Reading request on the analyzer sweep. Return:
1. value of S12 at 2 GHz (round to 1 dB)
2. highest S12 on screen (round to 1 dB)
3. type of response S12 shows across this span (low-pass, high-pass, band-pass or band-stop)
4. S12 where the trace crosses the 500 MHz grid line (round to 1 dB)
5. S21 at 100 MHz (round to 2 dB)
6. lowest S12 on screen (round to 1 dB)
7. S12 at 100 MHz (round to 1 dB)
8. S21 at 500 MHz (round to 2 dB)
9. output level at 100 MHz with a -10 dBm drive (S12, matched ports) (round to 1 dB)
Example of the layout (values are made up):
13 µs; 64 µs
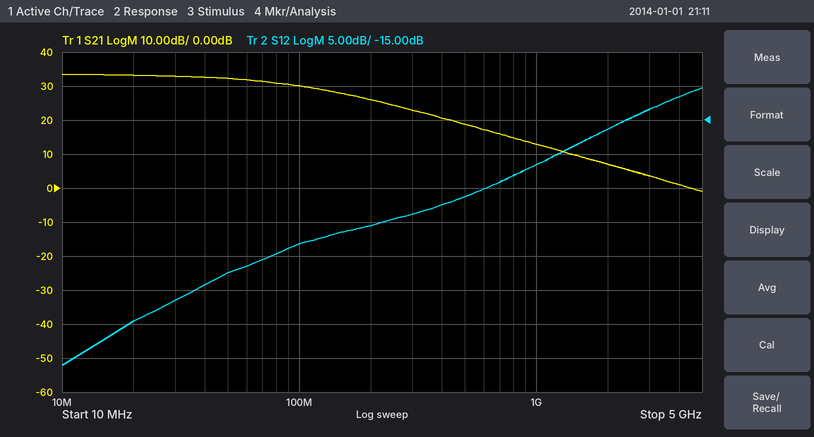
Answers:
-16 dB; -10 dB; high-pass; -26 dB; 30 dB; -51 dB; -33 dB; 18 dB; -43 dBm
